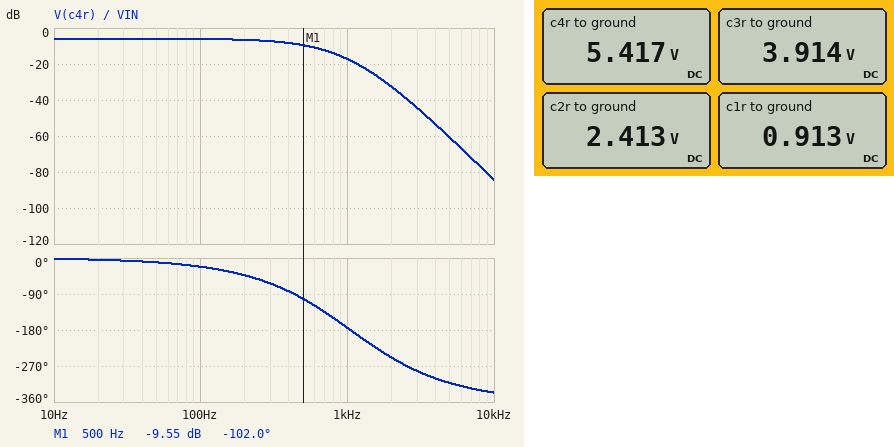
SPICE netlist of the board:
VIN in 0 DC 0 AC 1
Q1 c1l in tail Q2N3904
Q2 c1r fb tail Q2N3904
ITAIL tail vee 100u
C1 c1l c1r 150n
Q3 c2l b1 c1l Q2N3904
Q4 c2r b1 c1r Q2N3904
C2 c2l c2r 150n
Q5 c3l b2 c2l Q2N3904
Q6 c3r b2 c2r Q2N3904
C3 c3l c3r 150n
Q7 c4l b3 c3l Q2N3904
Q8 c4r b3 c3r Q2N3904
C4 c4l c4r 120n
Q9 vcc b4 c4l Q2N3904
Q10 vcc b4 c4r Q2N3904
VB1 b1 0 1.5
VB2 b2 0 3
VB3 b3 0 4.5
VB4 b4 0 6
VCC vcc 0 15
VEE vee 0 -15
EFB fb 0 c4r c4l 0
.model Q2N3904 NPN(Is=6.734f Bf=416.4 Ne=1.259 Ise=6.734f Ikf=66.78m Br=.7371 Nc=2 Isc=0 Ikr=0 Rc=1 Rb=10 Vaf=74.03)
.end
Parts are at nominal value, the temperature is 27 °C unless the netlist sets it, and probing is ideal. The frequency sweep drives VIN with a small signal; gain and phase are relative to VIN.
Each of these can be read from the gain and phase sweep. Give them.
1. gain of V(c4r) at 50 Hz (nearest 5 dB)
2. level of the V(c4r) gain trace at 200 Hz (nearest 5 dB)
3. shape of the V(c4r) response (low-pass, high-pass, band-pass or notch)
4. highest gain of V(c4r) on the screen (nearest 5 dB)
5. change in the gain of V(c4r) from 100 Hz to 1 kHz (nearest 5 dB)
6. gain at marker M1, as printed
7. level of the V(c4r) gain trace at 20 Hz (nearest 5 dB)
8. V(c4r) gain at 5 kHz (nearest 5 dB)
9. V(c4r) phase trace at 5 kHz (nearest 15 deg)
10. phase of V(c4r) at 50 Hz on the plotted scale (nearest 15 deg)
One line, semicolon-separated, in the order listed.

-5 dB; -5 dB; low-pass; -5 dB; -10 dB; -9.55 dB; -5 dB; -60 dB; -315 deg; -15 deg
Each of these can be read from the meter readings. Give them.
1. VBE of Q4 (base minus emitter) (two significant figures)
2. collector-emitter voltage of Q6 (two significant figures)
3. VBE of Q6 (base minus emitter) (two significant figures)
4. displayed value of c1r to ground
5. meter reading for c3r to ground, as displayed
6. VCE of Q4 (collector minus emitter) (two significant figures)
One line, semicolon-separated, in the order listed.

590 mV; 1.5 V; 590 mV; 0.913 V; 3.914 V; 1.5 V
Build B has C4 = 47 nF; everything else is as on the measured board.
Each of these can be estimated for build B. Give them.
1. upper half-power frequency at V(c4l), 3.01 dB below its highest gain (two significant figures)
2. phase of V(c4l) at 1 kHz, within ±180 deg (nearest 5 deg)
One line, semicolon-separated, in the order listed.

500 Hz; 25 deg
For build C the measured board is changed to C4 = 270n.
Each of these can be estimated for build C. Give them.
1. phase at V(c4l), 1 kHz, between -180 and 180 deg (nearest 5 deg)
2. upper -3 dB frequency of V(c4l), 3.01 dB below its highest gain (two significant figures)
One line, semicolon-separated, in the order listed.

-15 deg; 350 Hz
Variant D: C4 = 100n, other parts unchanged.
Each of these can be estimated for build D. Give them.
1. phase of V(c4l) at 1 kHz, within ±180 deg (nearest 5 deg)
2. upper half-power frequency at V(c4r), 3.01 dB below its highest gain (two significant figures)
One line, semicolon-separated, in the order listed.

10 deg; 470 Hz
